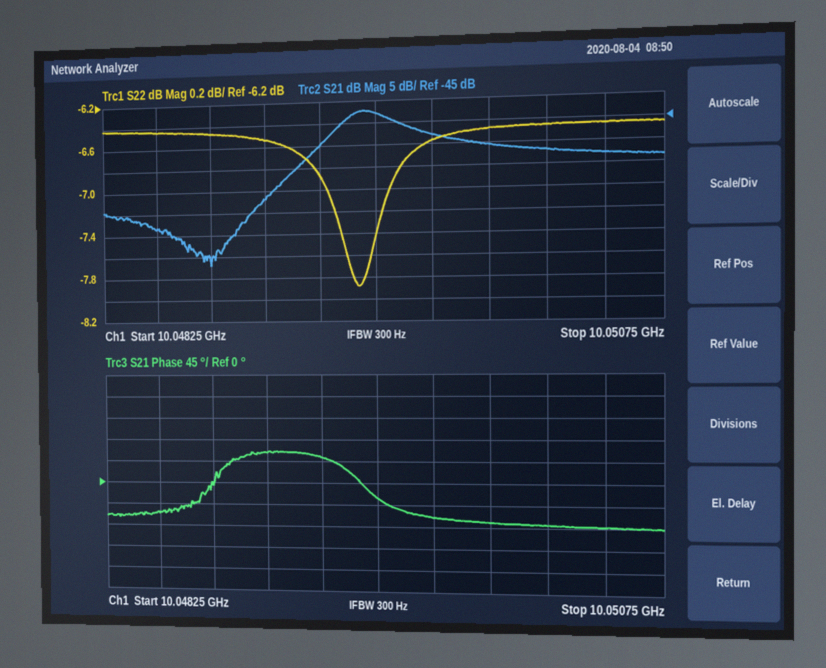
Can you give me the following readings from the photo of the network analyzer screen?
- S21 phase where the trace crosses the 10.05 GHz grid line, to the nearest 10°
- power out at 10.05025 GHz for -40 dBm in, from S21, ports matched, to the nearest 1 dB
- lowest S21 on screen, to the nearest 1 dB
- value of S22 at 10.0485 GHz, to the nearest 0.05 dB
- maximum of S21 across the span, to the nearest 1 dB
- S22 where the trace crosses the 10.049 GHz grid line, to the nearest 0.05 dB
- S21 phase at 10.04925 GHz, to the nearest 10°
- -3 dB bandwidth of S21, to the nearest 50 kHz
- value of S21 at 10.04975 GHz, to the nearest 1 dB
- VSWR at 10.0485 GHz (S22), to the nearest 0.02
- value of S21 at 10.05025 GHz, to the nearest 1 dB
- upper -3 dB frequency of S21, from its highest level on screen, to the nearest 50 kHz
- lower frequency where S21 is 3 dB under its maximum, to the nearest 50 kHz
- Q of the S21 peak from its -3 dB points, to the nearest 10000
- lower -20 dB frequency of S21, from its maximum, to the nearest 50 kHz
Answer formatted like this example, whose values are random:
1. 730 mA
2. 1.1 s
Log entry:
1. -80°
2. -92 dBm
3. -77 dB
4. -6.45 dB
5. -42 dB
6. -6.55 dB
7. 50°
8. 250 kHz
9. -48 dB
10. 2.82
11. -52 dB
12. 10.04960 GHz
13. 10.04935 GHz
14. 40000
15. 10.04900 GHz
